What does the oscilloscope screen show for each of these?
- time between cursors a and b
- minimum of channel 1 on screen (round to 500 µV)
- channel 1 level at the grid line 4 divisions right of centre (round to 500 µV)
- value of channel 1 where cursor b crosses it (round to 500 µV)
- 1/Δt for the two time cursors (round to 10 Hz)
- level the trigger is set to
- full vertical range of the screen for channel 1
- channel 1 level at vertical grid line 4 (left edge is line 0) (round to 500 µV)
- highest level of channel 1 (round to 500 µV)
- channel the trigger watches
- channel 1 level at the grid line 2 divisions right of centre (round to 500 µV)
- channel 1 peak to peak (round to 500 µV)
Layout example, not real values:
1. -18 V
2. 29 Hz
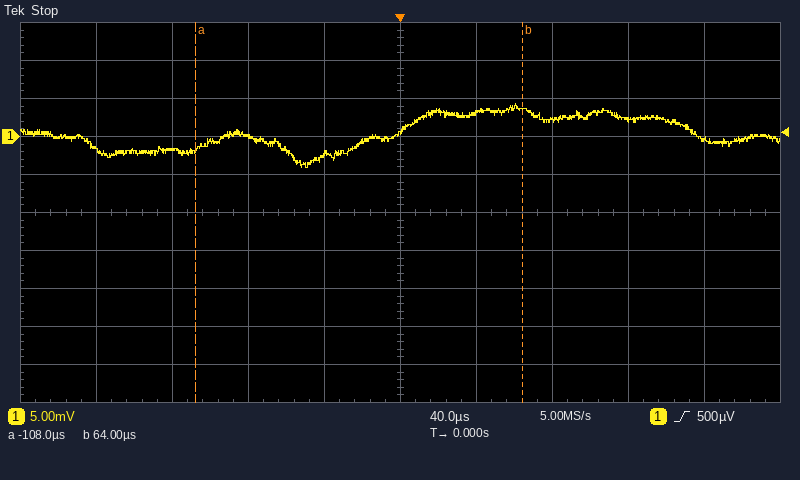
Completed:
1. 172 µs
2. -4.0 mV
3. -500 µV
4. 3.5 mV
5. 5.81 kHz
6. 500 µV
7. 50 mV
8. -2.5 mV
9. 4.5 mV
10. channel 1
11. 2.0 mV
12. 8.5 mV
